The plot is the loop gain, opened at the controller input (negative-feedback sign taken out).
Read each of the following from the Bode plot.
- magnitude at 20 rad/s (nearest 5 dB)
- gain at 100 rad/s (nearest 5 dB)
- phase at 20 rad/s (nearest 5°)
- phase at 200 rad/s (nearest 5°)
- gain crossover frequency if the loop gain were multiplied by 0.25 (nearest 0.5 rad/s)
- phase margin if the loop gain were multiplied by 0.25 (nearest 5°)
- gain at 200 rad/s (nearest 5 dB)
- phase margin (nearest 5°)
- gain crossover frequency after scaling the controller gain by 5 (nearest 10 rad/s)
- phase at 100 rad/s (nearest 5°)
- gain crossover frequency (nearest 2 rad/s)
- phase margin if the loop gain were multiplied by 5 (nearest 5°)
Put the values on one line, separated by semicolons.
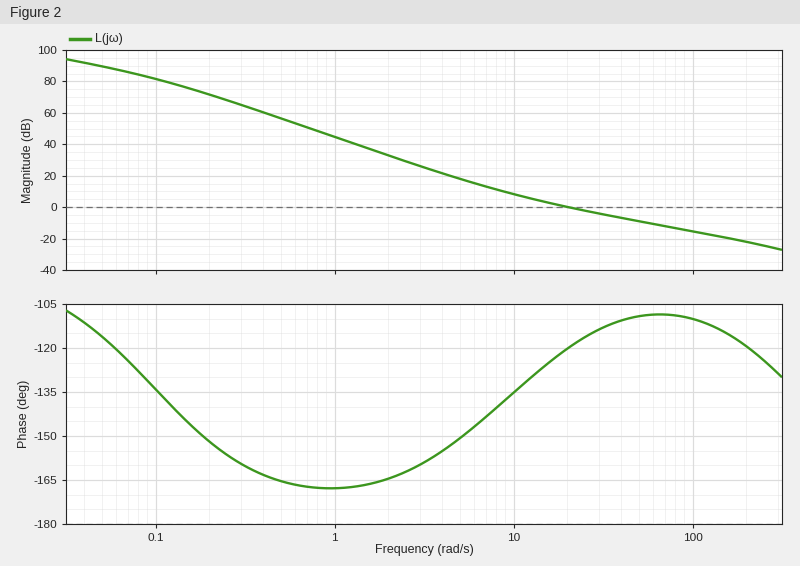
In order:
0 dB; -15 dB; -120°; -120°; 7.5 rad/s; 40°; -20 dB; 60°; 90 rad/s; -110°; 20 rad/s; 70°
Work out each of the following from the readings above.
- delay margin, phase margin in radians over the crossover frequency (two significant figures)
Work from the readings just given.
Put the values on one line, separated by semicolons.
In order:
0.052 s
